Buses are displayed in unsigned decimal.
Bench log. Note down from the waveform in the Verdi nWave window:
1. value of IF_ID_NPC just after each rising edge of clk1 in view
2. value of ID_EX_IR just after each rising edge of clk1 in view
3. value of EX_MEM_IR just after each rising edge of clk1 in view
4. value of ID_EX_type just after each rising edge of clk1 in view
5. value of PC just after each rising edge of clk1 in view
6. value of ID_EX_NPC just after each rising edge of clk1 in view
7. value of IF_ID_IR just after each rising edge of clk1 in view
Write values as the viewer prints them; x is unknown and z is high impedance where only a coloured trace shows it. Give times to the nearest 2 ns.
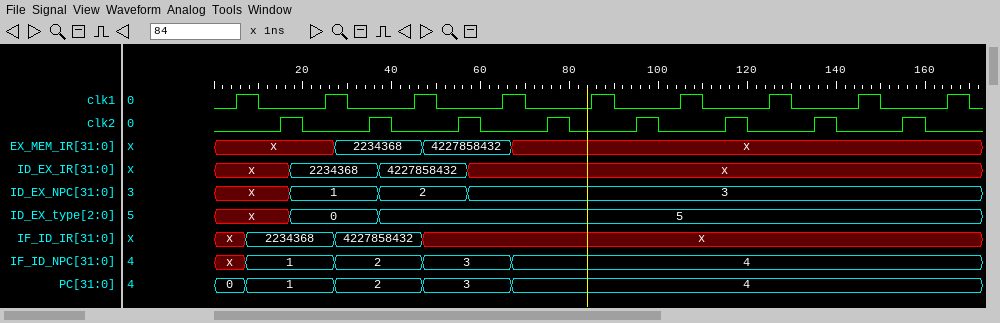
x, 1, 2, 3, 4, 4, 4, 4, 4
x, 2234368, 4227858432, x, x, x, x, x, x
x, x, 2234368, 4227858432, x, x, x, x, x
x, 0, 5, 5, 5, 5, 5, 5, 5
0, 1, 2, 3, 4, 4, 4, 4, 4
x, 1, 2, 3, 3, 3, 3, 3, 3
x, 2234368, 4227858432, x, x, x, x, x, x
